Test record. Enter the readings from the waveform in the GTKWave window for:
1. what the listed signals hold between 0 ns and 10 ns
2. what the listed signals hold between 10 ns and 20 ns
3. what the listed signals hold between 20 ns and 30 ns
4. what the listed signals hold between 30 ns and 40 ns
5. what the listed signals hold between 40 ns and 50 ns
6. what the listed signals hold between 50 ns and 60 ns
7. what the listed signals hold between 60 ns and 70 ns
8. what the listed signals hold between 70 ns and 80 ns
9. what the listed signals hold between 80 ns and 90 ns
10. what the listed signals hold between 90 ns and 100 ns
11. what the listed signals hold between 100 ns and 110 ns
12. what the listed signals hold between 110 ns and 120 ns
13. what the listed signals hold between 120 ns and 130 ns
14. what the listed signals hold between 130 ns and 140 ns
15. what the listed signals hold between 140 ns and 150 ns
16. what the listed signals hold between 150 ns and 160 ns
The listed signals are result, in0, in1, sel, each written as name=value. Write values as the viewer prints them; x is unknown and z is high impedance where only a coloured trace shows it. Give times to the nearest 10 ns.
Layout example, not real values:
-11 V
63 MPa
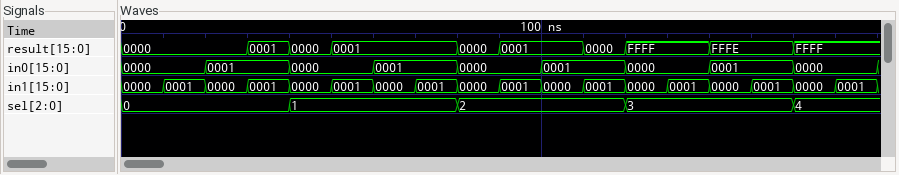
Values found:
result=0000, in0=0000, in1=0000, sel=0
result=0000, in0=0000, in1=0001, sel=0
result=0000, in0=0001, in1=0000, sel=0
result=0001, in0=0001, in1=0001, sel=0
result=0000, in0=0000, in1=0000, sel=1
result=0001, in0=0000, in1=0001, sel=1
result=0001, in0=0001, in1=0000, sel=1
result=0001, in0=0001, in1=0001, sel=1
result=0000, in0=0000, in1=0000, sel=2
result=0001, in0=0000, in1=0001, sel=2
result=0001, in0=0001, in1=0000, sel=2
result=0000, in0=0001, in1=0001, sel=2
result=FFFF, in0=0000, in1=0000, sel=3
result=FFFF, in0=0000, in1=0001, sel=3
result=FFFE, in0=0001, in1=0000, sel=3
result=FFFE, in0=0001, in1=0001, sel=3
